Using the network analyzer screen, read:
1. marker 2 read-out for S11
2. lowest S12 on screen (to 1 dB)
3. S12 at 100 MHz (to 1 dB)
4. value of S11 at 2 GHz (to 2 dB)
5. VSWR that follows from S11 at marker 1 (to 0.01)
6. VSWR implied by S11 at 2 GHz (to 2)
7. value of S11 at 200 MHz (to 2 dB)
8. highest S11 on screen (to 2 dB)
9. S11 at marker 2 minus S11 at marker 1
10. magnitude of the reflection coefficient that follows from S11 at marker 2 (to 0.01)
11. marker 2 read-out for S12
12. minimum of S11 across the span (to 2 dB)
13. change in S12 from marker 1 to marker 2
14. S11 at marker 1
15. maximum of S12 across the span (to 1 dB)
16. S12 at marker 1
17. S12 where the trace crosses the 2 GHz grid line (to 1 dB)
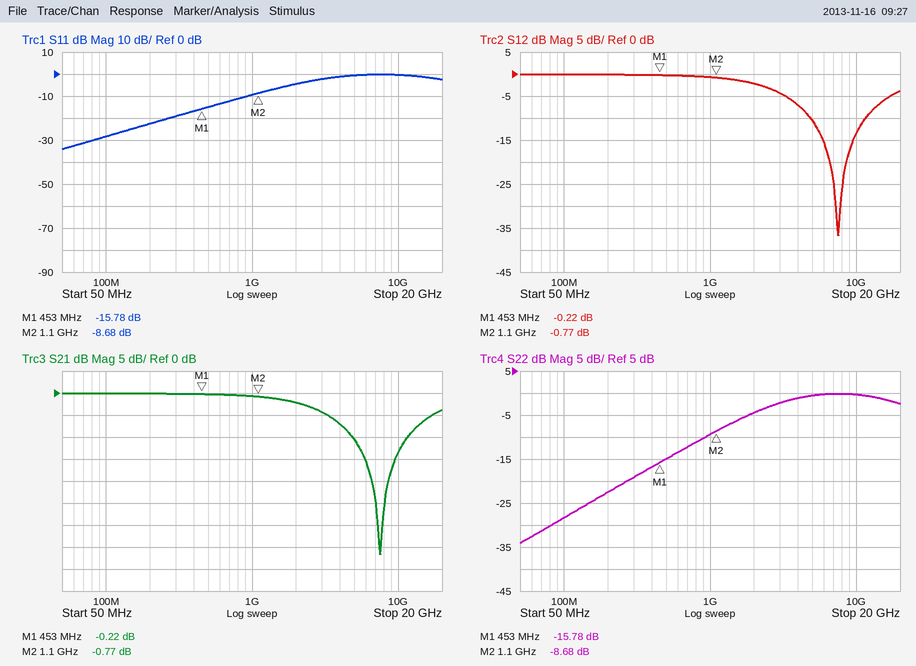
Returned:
-8.68 dB
-37 dB
0 dB
-4 dB
1.39
4
-22 dB
0 dB
7.10 dB
0.37
-0.77 dB
-34 dB
-0.55 dB
-15.78 dB
0 dB
-0.22 dB
-2 dB
